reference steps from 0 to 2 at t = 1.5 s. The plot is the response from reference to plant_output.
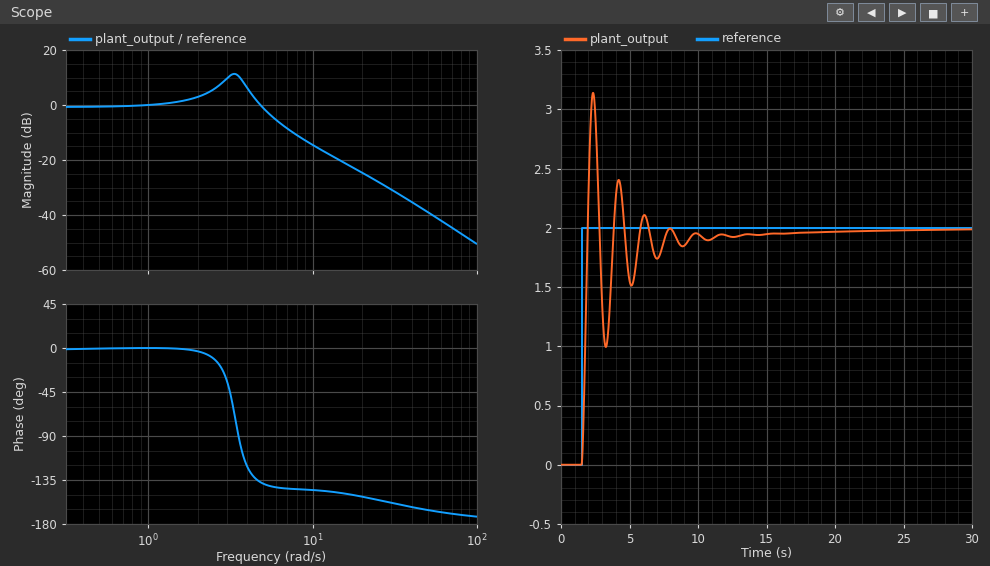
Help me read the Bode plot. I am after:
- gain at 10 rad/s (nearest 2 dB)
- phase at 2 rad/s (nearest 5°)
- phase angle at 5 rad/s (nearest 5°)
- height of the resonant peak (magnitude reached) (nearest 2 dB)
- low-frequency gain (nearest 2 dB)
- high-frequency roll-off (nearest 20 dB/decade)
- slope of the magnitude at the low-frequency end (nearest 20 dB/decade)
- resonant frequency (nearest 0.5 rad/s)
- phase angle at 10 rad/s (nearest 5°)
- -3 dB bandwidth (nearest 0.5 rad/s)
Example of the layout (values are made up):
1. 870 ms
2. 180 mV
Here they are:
1. -14 dB
2. -5°
3. -140°
4. 12 dB
5. 0 dB
6. -40 dB/decade
7. 0 dB/decade
8. 3.5 rad/s
9. -145°
10. 5.5 rad/s
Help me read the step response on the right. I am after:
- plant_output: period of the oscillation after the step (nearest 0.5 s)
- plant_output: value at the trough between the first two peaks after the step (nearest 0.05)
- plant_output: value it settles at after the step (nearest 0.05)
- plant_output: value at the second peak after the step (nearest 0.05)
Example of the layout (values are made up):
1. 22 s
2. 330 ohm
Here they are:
1. 2.0 s
2. 1.00
3. 2.00
4. 2.40
